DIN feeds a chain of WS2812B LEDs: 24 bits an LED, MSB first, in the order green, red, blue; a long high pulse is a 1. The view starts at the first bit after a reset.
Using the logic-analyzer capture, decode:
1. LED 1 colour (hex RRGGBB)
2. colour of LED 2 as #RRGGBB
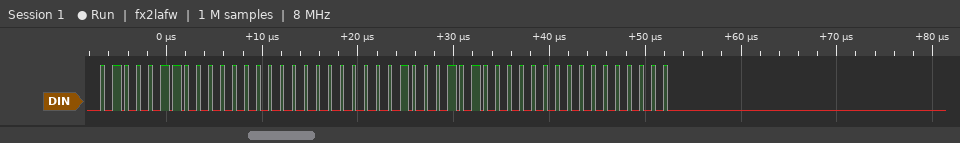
#004600
#004500
